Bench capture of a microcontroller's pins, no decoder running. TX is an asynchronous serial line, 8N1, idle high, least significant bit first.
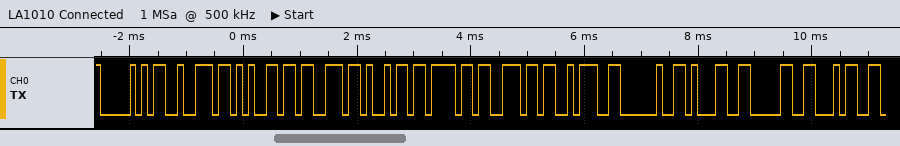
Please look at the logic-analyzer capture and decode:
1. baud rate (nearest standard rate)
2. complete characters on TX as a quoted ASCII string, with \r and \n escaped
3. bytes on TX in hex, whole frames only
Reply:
9600 baud
"Presion: 104"
50 72 65 73 69 6F 6E 3A 20 31 30 34
